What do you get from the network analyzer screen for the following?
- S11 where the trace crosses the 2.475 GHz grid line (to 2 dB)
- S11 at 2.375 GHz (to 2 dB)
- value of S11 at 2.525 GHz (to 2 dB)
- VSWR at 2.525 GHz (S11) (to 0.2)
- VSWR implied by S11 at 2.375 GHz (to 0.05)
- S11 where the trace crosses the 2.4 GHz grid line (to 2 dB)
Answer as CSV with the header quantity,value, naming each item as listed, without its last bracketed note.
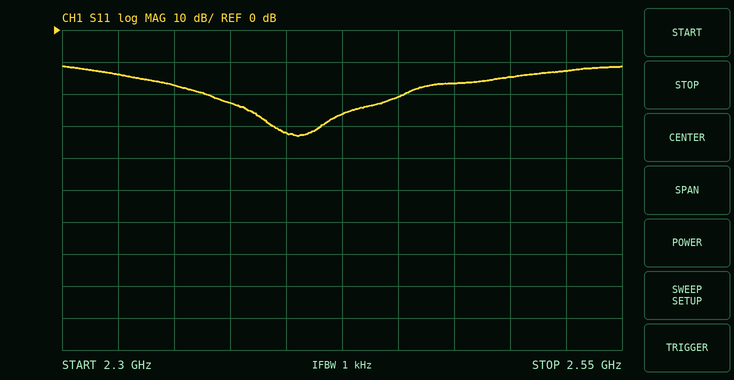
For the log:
quantity,value
S11 where the trace crosses the 2.475 GHz grid line,-16 dB
S11 at 2.375 GHz,-22 dB
value of S11 at 2.525 GHz,-12 dB
VSWR at 2.525 GHz (S11),1.6
VSWR implied by S11 at 2.375 GHz,1.15
S11 where the trace crosses the 2.4 GHz grid line,-32 dB
